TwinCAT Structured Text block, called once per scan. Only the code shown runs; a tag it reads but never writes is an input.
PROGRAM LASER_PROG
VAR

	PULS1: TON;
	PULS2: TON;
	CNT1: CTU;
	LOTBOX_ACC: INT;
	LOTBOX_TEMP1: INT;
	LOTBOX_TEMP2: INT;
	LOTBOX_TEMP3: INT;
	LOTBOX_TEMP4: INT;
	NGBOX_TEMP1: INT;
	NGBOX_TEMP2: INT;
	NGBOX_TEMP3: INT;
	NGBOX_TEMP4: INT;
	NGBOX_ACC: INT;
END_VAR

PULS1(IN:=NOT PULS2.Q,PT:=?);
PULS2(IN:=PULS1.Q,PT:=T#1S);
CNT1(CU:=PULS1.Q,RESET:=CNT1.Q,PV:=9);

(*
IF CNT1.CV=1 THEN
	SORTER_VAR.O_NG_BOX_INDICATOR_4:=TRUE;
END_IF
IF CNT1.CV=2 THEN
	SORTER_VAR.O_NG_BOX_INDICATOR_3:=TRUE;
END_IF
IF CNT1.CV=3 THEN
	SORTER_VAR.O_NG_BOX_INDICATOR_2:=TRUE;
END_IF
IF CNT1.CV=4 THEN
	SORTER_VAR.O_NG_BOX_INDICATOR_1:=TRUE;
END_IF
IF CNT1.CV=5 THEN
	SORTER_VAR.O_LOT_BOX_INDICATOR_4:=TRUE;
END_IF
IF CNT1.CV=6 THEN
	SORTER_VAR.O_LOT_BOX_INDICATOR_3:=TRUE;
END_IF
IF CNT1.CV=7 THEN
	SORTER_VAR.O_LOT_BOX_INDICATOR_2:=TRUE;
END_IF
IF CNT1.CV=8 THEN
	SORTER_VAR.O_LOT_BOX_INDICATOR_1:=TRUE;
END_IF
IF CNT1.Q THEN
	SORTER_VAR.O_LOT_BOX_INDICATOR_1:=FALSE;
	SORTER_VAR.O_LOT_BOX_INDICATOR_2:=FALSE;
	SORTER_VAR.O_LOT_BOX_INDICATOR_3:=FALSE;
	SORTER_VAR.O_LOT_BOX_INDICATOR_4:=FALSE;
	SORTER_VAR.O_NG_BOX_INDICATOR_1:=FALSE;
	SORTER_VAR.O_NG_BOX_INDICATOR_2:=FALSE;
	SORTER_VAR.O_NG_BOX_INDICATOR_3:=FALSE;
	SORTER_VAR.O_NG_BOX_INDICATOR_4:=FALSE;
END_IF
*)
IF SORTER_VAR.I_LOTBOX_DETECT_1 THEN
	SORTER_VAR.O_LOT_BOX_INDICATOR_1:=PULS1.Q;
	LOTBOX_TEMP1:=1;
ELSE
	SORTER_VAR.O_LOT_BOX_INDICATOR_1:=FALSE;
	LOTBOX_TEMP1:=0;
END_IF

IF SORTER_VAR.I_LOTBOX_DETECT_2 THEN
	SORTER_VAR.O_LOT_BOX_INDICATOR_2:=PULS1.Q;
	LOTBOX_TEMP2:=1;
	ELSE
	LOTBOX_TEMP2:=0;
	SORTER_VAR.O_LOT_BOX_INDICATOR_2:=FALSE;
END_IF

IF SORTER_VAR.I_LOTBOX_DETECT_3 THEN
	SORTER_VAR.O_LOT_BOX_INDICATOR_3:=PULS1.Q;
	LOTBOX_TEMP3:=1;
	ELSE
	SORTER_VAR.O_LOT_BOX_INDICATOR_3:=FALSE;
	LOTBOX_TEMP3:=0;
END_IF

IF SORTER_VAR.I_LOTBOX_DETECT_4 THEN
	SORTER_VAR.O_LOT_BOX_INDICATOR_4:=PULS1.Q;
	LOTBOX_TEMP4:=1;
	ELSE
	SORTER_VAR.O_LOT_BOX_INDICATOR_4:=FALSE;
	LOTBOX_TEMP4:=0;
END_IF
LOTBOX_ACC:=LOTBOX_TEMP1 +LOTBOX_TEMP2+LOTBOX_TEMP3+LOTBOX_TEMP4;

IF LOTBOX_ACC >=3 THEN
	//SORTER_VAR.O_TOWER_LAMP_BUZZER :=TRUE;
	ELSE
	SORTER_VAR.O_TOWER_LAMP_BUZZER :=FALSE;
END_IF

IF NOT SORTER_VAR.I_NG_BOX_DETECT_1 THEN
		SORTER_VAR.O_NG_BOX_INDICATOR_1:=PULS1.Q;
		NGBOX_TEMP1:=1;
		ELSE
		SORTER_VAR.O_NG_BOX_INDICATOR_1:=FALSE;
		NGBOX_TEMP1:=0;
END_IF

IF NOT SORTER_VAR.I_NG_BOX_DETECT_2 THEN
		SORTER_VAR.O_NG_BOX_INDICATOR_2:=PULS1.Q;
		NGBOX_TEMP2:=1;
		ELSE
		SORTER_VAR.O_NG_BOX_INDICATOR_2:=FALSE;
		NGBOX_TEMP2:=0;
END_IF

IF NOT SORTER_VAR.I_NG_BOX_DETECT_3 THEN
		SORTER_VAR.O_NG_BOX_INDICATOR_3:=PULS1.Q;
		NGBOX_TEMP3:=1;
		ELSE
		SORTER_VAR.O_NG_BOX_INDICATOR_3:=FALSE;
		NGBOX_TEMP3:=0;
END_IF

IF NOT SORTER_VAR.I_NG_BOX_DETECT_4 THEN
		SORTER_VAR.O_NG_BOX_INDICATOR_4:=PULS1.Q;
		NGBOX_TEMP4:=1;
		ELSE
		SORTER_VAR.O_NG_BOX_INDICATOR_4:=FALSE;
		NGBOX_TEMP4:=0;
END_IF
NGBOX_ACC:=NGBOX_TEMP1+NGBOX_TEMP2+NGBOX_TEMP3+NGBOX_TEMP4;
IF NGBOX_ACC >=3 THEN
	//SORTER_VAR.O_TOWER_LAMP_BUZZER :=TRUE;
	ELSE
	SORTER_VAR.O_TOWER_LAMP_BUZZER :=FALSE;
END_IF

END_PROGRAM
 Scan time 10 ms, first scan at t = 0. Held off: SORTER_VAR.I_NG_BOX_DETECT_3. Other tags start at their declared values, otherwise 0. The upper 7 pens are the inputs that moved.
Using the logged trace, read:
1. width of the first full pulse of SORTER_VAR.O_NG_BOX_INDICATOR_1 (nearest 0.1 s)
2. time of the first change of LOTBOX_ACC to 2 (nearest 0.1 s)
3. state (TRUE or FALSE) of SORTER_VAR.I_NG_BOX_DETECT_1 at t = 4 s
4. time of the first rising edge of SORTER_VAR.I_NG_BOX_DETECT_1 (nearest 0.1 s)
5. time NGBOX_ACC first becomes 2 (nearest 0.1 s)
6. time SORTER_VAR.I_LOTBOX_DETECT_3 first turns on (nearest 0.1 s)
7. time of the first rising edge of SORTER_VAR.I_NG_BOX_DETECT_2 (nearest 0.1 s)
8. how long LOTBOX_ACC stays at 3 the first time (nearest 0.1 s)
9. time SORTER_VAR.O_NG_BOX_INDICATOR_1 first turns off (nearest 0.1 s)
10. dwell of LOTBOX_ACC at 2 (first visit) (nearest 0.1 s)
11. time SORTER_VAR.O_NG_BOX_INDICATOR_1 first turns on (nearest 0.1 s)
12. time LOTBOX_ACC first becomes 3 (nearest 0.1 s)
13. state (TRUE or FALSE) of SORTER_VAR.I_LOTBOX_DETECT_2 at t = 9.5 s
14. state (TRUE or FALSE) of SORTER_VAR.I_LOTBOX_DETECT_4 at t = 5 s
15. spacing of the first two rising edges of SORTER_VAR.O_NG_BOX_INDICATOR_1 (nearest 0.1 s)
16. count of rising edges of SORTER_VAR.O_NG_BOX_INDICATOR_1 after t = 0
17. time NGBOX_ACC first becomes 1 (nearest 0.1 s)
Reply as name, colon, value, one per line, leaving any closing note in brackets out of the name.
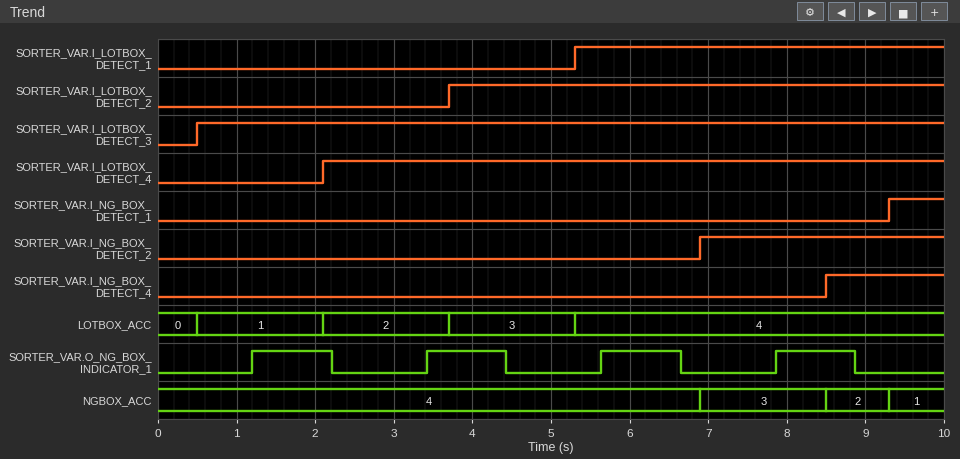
width of the first full pulse of SORTER_VAR.O_NG_BOX_INDICATOR_1: 1.0 s
time of the first change of LOTBOX_ACC to 2: 2.1 s
state (TRUE or FALSE) of SORTER_VAR.I_NG_BOX_DETECT_1 at t = 4 s: FALSE
time of the first rising edge of SORTER_VAR.I_NG_BOX_DETECT_1: 9.3 s
time NGBOX_ACC first becomes 2: 8.5 s
time SORTER_VAR.I_LOTBOX_DETECT_3 first turns on: 0.5 s
time of the first rising edge of SORTER_VAR.I_NG_BOX_DETECT_2: 6.9 s
how long LOTBOX_ACC stays at 3 the first time: 1.6 s
time SORTER_VAR.O_NG_BOX_INDICATOR_1 first turns off: 2.2 s
dwell of LOTBOX_ACC at 2 (first visit): 1.6 s
time SORTER_VAR.O_NG_BOX_INDICATOR_1 first turns on: 1.2 s
time LOTBOX_ACC first becomes 3: 3.7 s
state (TRUE or FALSE) of SORTER_VAR.I_LOTBOX_DETECT_2 at t = 9.5 s: TRUE
state (TRUE or FALSE) of SORTER_VAR.I_LOTBOX_DETECT_4 at t = 5 s: TRUE
spacing of the first two rising edges of SORTER_VAR.O_NG_BOX_INDICATOR_1: 2.2 s
count of rising edges of SORTER_VAR.O_NG_BOX_INDICATOR_1 after t = 0: 4
time NGBOX_ACC first becomes 1: 9.3 s
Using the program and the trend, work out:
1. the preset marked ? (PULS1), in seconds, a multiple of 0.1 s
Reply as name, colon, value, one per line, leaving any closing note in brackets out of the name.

the preset marked ? (PULS1), in seconds, a multiple of 0.1 s: 1.2 s
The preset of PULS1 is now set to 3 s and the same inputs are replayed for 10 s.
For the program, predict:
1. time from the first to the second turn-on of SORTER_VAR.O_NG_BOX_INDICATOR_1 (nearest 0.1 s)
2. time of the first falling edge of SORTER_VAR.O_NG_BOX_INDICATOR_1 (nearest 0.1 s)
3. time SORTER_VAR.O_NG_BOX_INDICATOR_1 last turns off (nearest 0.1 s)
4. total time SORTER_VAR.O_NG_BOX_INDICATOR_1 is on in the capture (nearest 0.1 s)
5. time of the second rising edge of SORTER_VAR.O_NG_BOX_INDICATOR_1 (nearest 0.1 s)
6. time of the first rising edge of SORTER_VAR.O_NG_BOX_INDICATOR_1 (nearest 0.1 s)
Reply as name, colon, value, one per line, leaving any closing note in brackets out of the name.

time from the first to the second turn-on of SORTER_VAR.O_NG_BOX_INDICATOR_1: 4.0 s
time of the first falling edge of SORTER_VAR.O_NG_BOX_INDICATOR_1: 4.0 s
time SORTER_VAR.O_NG_BOX_INDICATOR_1 last turns off: 8.0 s
total time SORTER_VAR.O_NG_BOX_INDICATOR_1 is on in the capture: 2.0 s
time of the second rising edge of SORTER_VAR.O_NG_BOX_INDICATOR_1: 7.0 s
time of the first rising edge of SORTER_VAR.O_NG_BOX_INDICATOR_1: 3.0 s
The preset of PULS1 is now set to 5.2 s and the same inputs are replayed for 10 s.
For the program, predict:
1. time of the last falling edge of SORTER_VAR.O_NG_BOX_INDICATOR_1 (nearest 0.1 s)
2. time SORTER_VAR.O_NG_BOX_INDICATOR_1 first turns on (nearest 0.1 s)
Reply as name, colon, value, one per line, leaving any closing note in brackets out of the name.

time of the last falling edge of SORTER_VAR.O_NG_BOX_INDICATOR_1: 6.2 s
time SORTER_VAR.O_NG_BOX_INDICATOR_1 first turns on: 5.2 s
